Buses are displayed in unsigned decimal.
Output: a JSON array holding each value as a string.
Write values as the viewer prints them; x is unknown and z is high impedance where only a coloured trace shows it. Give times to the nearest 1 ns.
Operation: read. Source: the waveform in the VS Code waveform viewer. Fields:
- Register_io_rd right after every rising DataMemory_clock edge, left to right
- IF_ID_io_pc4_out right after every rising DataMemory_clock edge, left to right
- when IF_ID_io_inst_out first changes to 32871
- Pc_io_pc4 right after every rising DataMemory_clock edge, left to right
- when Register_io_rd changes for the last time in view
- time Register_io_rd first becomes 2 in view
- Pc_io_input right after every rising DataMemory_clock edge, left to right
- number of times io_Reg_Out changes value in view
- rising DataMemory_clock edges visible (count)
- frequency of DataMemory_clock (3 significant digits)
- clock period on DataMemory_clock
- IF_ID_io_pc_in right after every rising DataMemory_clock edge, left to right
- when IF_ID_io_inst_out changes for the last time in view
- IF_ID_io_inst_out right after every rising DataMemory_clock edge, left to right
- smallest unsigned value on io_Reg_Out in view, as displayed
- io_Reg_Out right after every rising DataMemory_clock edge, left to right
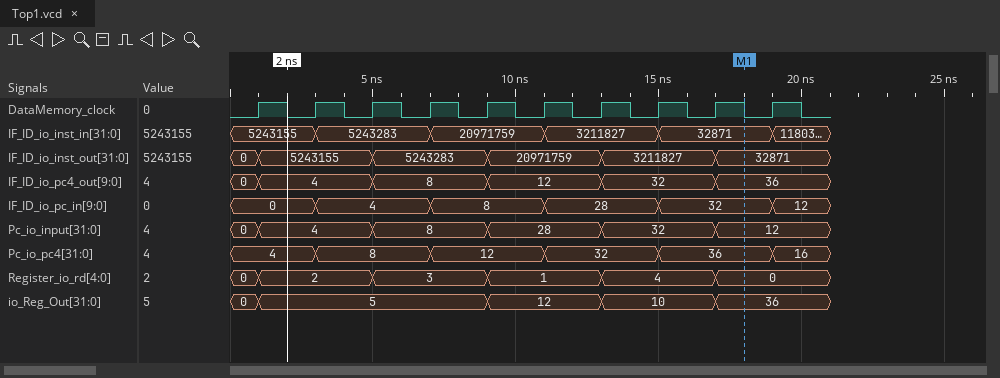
["2, 2, 3, 3, 1, 1, 4, 4, 0, 0", "4, 4, 8, 8, 12, 12, 32, 32, 36, 36", "17 ns", "4, 8, 8, 12, 12, 32, 32, 36, 36, 16", "17 ns", "1 ns", "4, 4, 8, 8, 28, 28, 32, 32, 12, 12", "4", "10", "500 MHz", "2 ns", "0, 4, 4, 8, 8, 28, 28, 32, 32, 12", "17 ns", "5243155, 5243155, 5243283, 5243283, 20971759, 20971759, 3211827, 3211827, 32871, 32871", "0", "5, 5, 5, 5, 12, 12, 10, 10, 36, 36"]
